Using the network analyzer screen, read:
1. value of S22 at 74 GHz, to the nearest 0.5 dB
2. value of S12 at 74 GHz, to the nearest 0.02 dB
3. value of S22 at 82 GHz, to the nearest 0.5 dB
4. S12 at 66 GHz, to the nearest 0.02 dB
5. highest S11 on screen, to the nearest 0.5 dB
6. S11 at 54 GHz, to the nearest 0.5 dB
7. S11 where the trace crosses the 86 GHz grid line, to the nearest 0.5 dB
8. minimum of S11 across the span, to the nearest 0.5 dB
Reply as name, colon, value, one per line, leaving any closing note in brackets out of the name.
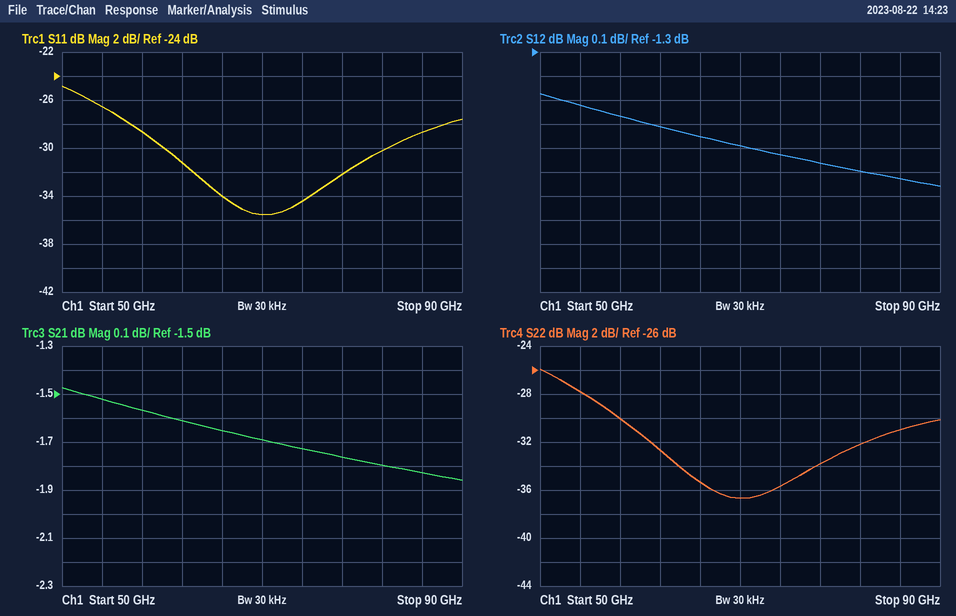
value of S22 at 74 GHz, to the nearest 0.5 dB: -35.5 dB
value of S12 at 74 GHz, to the nearest 0.02 dB: -1.72 dB
value of S22 at 82 GHz, to the nearest 0.5 dB: -32.0 dB
S12 at 66 GHz, to the nearest 0.02 dB: -1.66 dB
highest S11 on screen, to the nearest 0.5 dB: -25.0 dB
S11 at 54 GHz, to the nearest 0.5 dB: -26.5 dB
S11 where the trace crosses the 86 GHz grid line, to the nearest 0.5 dB: -28.5 dB
minimum of S11 across the span, to the nearest 0.5 dB: -35.5 dB
